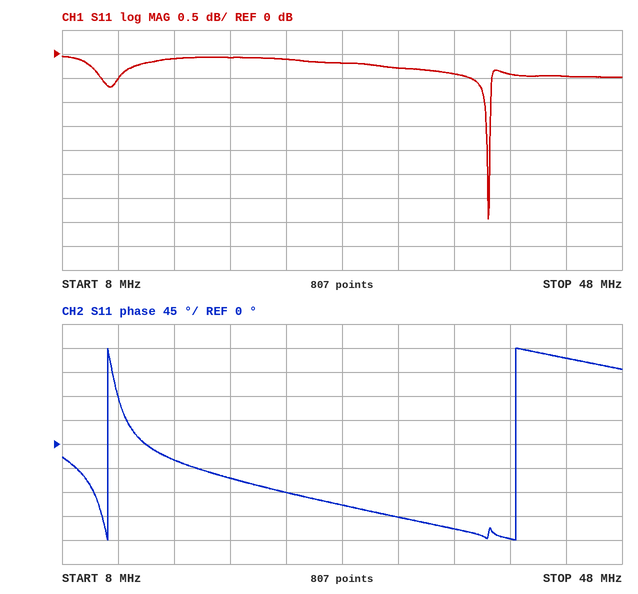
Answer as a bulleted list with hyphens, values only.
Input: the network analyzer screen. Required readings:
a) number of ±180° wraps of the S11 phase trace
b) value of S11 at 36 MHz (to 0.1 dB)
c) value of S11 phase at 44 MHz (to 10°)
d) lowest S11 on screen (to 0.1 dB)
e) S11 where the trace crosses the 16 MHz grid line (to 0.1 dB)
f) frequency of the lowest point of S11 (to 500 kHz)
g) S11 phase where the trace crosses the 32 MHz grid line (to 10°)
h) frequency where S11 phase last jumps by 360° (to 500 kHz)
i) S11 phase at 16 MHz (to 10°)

- 2
- -0.4 dB
- 160°
- -3.4 dB
- -0.1 dB
- 38.5 MHz
- -140°
- 40.5 MHz
- -30°
